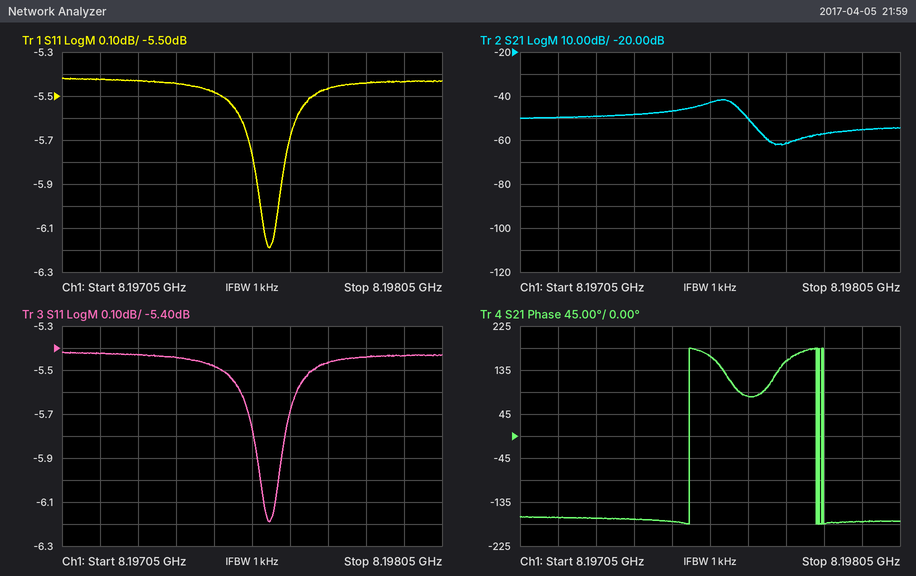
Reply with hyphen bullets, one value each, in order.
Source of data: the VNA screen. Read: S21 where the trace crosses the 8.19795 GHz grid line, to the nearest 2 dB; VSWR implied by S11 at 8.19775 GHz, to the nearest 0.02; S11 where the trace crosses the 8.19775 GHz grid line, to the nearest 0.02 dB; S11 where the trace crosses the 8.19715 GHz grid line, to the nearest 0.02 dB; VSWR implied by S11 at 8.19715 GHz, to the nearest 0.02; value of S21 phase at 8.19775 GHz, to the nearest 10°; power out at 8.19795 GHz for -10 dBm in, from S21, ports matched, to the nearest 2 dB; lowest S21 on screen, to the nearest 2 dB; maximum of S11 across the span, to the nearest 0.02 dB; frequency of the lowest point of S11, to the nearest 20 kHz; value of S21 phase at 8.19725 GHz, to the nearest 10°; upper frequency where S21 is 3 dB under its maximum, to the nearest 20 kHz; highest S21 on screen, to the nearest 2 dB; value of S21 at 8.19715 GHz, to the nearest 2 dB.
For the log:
- -56 dB
- 3.28
- -5.46 dB
- -5.42 dB
- 3.30
- 150°
- -66 dBm
- -62 dB
- -5.42 dB
- 8.19760 GHz
- -170°
- 8.19762 GHz
- -42 dB
- -50 dB
